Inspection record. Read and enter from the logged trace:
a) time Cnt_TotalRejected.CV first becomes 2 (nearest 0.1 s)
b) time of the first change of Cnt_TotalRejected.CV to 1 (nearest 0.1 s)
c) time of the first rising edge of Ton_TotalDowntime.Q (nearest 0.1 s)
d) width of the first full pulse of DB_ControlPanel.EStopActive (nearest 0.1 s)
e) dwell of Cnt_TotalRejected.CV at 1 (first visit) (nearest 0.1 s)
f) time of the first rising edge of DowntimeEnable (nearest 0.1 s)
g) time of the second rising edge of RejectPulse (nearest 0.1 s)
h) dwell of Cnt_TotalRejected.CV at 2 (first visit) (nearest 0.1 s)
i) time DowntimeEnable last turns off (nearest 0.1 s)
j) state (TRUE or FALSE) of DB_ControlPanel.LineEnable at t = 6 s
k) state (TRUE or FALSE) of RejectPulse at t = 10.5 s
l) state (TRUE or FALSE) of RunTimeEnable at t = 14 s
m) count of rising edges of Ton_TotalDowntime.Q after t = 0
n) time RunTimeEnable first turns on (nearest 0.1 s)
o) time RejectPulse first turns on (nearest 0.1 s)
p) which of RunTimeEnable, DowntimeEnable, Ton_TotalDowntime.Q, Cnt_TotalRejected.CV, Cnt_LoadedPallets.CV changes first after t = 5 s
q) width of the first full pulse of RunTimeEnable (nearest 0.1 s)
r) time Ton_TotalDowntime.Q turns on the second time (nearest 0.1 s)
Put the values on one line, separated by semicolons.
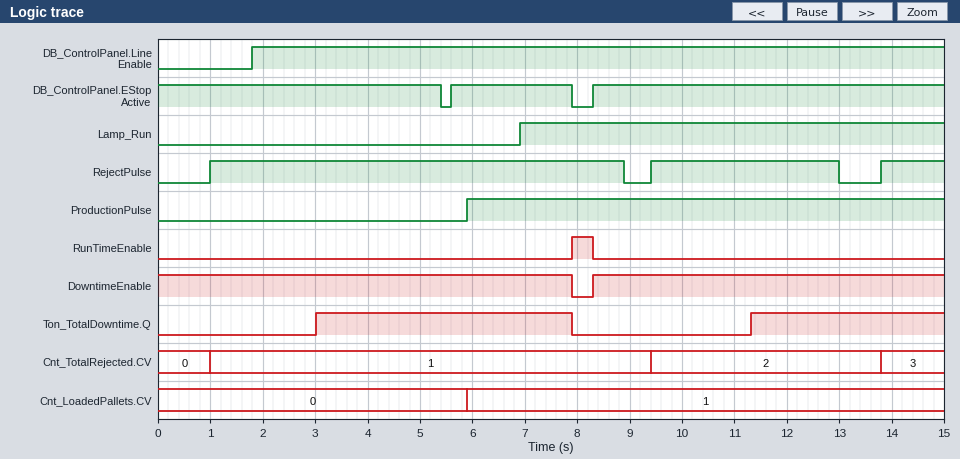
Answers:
9.4 s; 1.0 s; 3.0 s; 2.3 s; 8.4 s; 8.3 s; 9.4 s; 4.4 s; 7.9 s; TRUE; TRUE; FALSE; 2; 7.9 s; 1.0 s; Cnt_LoadedPallets.CV; 0.4 s; 11.3 s
